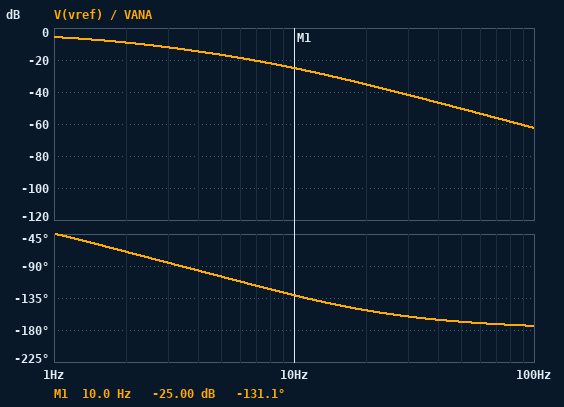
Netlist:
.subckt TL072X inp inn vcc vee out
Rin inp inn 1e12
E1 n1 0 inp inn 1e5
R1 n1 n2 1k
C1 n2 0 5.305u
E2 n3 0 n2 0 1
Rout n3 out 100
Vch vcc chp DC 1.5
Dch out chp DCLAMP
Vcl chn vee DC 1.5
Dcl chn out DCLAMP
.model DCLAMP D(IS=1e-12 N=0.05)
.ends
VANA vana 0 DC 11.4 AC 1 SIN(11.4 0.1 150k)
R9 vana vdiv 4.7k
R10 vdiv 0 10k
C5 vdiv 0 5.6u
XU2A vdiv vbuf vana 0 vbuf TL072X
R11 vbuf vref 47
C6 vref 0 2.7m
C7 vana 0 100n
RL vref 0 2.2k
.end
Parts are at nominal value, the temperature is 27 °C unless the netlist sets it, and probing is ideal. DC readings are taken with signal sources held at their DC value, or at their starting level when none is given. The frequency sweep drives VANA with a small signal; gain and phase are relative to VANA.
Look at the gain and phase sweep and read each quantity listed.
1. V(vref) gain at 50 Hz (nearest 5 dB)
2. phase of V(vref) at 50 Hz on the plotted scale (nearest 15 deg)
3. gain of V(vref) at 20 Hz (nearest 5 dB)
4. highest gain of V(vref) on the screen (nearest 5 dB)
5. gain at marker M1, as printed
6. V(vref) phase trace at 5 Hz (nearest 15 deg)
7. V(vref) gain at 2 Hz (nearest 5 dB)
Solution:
-50 dB
-165 deg
-35 dB
-5 dB
-25.00 dB
-105 deg
-10 dB
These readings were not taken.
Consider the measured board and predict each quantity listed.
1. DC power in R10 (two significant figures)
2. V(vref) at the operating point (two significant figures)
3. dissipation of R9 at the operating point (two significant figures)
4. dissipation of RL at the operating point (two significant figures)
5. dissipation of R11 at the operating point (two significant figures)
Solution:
6.0 mW
7.6 V
2.8 mW
26 mW
560 µW
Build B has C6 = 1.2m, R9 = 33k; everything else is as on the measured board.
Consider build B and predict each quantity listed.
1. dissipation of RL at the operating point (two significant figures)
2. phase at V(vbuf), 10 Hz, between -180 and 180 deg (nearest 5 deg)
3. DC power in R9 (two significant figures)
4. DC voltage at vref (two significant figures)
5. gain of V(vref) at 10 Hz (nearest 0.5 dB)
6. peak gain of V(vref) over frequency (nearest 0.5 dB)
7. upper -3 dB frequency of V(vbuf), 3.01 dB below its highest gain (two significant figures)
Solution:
3.1 mW
-70 deg
2.3 mW
2.6 V
-33.0 dB
-13.0 dB
3.7 Hz
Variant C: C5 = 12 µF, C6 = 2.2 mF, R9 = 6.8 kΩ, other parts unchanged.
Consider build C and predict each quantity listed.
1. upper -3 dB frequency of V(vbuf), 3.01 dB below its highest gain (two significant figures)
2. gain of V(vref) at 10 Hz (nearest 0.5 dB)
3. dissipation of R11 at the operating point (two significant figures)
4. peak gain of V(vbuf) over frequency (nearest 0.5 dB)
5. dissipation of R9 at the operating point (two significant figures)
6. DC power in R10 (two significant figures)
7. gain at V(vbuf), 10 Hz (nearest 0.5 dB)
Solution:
3.3 Hz
-31.0 dB
430 µW
-4.5 dB
3.1 mW
4.6 mW
-14.5 dB
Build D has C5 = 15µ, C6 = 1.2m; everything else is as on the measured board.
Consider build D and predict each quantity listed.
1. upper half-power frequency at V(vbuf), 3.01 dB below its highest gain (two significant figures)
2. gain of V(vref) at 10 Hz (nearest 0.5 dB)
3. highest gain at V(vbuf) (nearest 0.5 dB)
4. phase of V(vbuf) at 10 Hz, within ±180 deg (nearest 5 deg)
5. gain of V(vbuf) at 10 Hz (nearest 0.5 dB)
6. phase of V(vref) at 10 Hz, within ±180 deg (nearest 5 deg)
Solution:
3.3 Hz
-24.5 dB
-3.5 dB
-70 deg
-13.5 dB
-145 deg
